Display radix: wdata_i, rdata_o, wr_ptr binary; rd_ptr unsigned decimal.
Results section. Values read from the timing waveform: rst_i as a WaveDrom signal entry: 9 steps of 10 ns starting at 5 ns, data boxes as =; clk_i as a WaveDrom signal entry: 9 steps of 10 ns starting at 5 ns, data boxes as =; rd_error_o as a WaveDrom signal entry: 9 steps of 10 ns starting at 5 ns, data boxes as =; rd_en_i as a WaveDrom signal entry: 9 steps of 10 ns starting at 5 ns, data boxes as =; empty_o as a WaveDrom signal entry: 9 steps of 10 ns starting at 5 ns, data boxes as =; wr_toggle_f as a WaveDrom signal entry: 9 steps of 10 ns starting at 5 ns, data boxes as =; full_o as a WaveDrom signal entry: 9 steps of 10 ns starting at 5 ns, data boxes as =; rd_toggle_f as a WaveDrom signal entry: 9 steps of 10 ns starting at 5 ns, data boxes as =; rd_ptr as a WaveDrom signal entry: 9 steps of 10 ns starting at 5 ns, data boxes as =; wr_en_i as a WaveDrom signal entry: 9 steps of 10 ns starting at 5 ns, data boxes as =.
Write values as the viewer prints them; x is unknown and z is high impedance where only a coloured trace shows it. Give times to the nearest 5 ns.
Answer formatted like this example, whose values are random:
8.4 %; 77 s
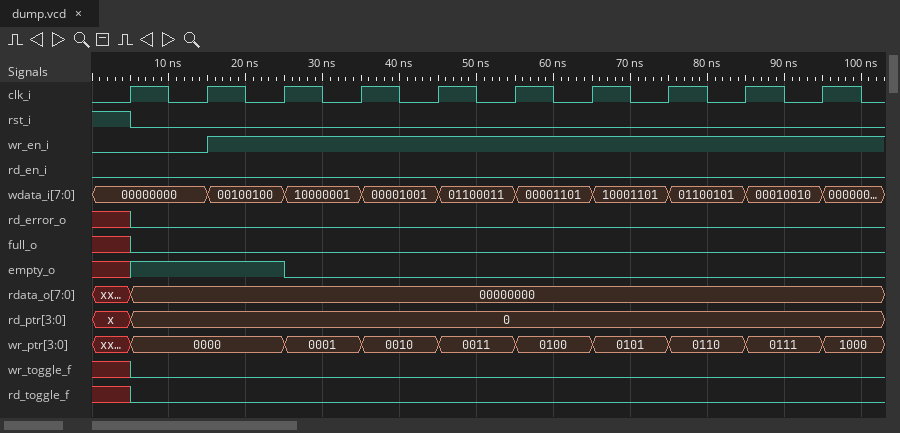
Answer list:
{name: 'rst_i', wave: '0........'}; {name: 'clk_i', wave: 'p........'}; {name: 'rd_error_o', wave: '0........'}; {name: 'rd_en_i', wave: '0........'}; {name: 'empty_o', wave: '1.0......'}; {name: 'wr_toggle_f', wave: '0........'}; {name: 'full_o', wave: '0........'}; {name: 'rd_toggle_f', wave: '0........'}; {name: 'rd_ptr', wave: '=........', data: '0'}; {name: 'wr_en_i', wave: '01.......'}
